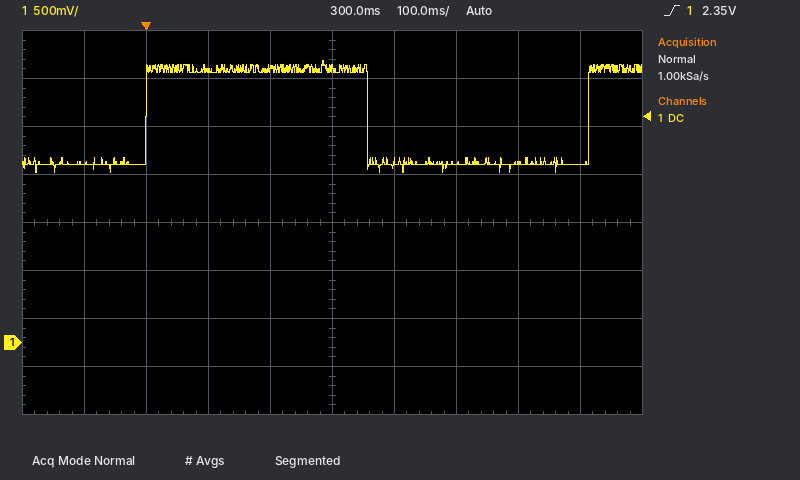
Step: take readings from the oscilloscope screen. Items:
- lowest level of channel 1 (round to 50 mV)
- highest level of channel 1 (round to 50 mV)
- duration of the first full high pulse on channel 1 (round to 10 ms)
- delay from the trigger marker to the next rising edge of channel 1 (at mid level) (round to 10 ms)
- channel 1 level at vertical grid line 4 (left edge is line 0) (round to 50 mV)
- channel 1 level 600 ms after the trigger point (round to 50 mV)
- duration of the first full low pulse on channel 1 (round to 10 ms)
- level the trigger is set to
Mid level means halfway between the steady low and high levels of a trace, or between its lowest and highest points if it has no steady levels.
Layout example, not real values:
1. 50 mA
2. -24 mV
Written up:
1. 1.75 V
2. 2.95 V
3. 360 ms
4. 710 ms
5. 2.85 V
6. 1.85 V
7. 360 ms
8. 2.35 V
